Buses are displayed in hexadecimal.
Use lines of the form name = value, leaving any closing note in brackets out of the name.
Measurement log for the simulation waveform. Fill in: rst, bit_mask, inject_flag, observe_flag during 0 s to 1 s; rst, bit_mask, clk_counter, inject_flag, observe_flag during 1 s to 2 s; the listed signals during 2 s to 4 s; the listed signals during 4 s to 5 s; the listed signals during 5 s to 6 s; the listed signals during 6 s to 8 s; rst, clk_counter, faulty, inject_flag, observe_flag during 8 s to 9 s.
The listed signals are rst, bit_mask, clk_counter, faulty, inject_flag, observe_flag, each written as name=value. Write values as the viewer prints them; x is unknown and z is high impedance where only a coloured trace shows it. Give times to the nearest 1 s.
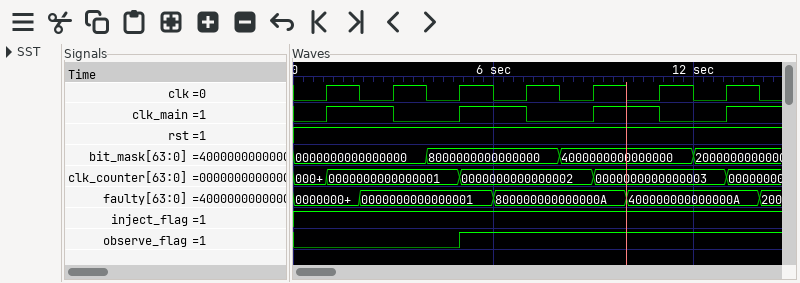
rst, bit_mask, inject_flag, observe_flag during 0 s to 1 s = rst=1, bit_mask=0000000000000000, inject_flag=1, observe_flag=0
rst, bit_mask, clk_counter, inject_flag, observe_flag during 1 s to 2 s = rst=1, bit_mask=0000000000000000, clk_counter=0000000000000001, inject_flag=1, observe_flag=0
the listed signals during 2 s to 4 s = rst=1, bit_mask=0000000000000000, clk_counter=0000000000000001, faulty=0000000000000001, inject_flag=1, observe_flag=0
the listed signals during 4 s to 5 s = rst=1, bit_mask=8000000000000000, clk_counter=0000000000000001, faulty=0000000000000001, inject_flag=1, observe_flag=0
the listed signals during 5 s to 6 s = rst=1, bit_mask=8000000000000000, clk_counter=0000000000000002, faulty=0000000000000001, inject_flag=1, observe_flag=1
the listed signals during 6 s to 8 s = rst=1, bit_mask=8000000000000000, clk_counter=0000000000000002, faulty=800000000000000A, inject_flag=1, observe_flag=1
rst, clk_counter, faulty, inject_flag, observe_flag during 8 s to 9 s = rst=1, clk_counter=0000000000000002, faulty=800000000000000A, inject_flag=1, observe_flag=1
